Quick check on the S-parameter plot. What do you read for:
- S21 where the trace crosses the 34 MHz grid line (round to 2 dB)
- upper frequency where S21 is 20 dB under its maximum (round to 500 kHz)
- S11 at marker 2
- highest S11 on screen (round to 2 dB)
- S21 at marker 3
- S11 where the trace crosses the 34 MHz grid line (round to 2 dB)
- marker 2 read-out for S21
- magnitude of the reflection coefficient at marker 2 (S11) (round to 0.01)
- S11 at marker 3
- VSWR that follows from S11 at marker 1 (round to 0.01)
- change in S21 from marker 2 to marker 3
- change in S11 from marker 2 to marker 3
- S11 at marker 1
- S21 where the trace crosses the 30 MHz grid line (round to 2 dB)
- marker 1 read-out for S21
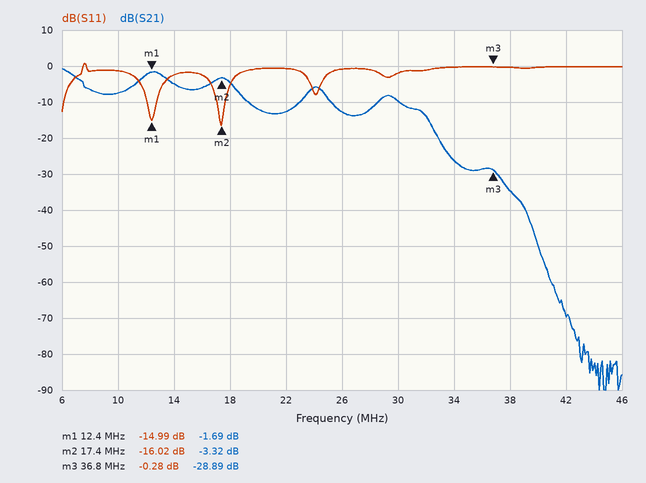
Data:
-26 dB
33.0 MHz
-16.02 dB
0 dB
-28.89 dB
0 dB
-3.32 dB
0.16
-0.28 dB
1.43
-25.57 dB
15.74 dB
-14.99 dB
-10 dB
-1.69 dB
